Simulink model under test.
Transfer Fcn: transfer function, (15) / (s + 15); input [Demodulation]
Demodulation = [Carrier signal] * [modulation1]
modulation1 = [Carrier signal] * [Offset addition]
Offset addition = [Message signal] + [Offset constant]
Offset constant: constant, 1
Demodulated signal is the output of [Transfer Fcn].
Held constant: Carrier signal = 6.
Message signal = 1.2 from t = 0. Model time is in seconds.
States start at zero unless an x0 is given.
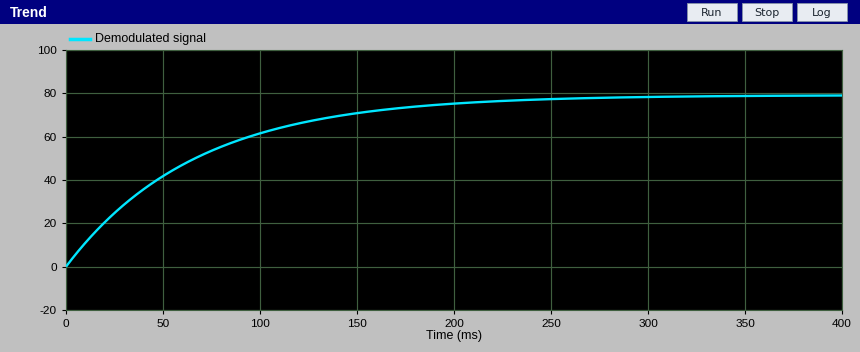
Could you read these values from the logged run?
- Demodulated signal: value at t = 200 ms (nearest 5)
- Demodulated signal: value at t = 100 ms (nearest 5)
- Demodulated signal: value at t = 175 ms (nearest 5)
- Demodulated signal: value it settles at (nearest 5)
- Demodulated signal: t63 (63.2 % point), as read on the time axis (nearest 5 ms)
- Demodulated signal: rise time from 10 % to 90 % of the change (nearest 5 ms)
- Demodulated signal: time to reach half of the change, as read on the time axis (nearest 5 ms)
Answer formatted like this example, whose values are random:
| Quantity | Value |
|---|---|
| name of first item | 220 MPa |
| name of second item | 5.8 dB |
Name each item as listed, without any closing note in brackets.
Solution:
| Quantity | Value |
|---|---|
| Demodulated signal: value at t = 200 ms | 75 |
| Demodulated signal: value at t = 100 ms | 60 |
| Demodulated signal: value at t = 175 ms | 75 |
| Demodulated signal: value it settles at | 80 |
| Demodulated signal: t63 (63.2 % point), as read on the time axis | 65 ms |
| Demodulated signal: rise time from 10 % to 90 % of the change | 145 ms |
| Demodulated signal: time to reach half of the change, as read on the time axis | 45 ms |
